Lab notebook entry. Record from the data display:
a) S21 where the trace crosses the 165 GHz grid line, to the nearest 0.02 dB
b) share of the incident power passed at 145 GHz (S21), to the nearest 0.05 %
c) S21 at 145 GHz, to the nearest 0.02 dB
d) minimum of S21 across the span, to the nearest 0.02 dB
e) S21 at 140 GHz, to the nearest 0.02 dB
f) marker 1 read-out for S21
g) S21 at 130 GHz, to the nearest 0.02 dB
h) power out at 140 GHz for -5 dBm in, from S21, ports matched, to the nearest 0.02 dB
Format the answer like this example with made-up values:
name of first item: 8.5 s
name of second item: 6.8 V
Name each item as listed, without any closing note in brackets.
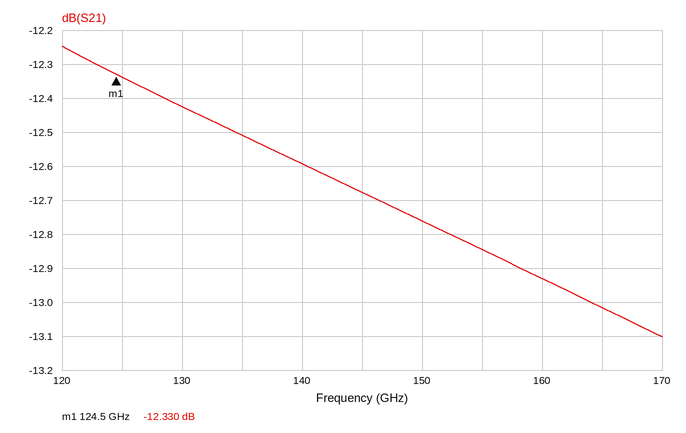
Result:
S21 where the trace crosses the 165 GHz grid line, to the nearest 0.02 dB: -13.02 dB
share of the incident power passed at 145 GHz (S21), to the nearest 0.05 %: 5.40 %
S21 at 145 GHz, to the nearest 0.02 dB: -12.68 dB
minimum of S21 across the span, to the nearest 0.02 dB: -13.10 dB
S21 at 140 GHz, to the nearest 0.02 dB: -12.60 dB
marker 1 read-out for S21: -12.330 dB
S21 at 130 GHz, to the nearest 0.02 dB: -12.42 dB
power out at 140 GHz for -5 dBm in, from S21, ports matched, to the nearest 0.02 dB: -17.60 dBm
